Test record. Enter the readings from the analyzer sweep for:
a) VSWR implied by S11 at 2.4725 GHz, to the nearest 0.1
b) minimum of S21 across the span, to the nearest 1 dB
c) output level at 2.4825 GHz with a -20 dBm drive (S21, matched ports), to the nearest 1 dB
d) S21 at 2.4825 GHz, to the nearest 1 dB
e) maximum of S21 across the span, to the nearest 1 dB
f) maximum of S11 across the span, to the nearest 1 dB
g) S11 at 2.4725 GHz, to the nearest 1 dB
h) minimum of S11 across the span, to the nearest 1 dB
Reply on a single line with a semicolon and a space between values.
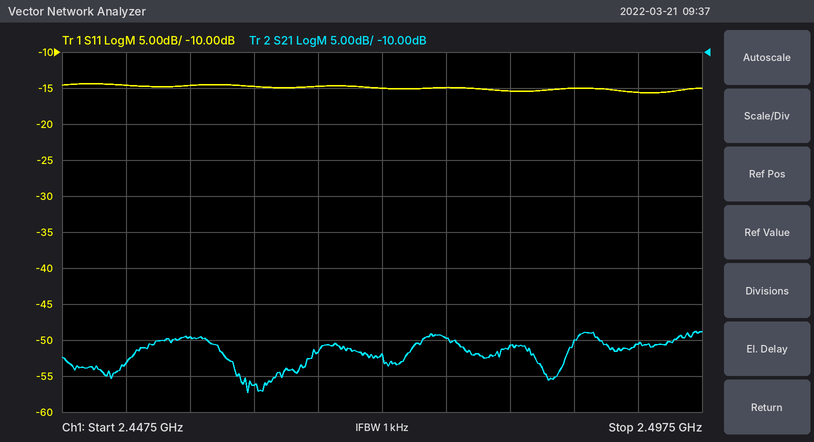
1.4; -57 dB; -71 dBm; -51 dB; -49 dB; -14 dB; -15 dB; -16 dB
